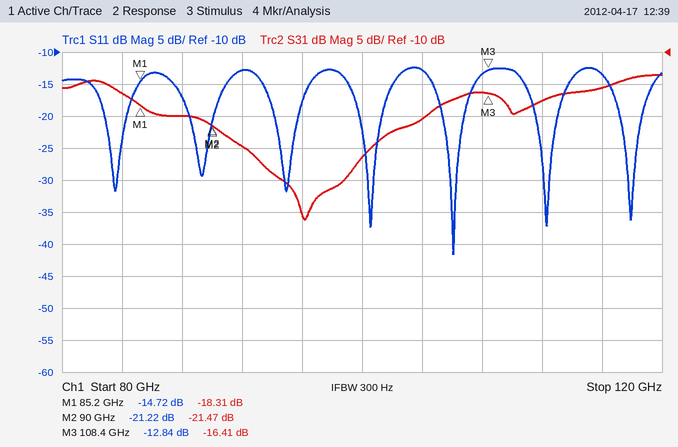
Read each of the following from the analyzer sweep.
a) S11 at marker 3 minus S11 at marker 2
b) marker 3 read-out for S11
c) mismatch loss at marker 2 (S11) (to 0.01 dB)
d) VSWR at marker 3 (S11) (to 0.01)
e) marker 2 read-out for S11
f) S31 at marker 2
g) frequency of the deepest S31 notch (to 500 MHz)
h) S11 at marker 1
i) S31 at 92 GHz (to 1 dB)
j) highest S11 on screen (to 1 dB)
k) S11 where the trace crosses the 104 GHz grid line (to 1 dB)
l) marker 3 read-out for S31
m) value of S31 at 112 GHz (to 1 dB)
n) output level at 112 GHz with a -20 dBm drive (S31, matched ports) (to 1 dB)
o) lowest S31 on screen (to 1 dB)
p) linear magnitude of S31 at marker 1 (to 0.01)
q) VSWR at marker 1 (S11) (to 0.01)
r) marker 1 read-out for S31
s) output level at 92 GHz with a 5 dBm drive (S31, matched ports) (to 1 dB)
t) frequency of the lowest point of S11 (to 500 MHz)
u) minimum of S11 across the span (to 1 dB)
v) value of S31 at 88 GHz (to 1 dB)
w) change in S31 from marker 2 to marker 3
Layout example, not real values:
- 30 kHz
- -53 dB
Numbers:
- 8.38 dB
- -12.84 dB
- 0.03 dB
- 1.59
- -21.22 dB
- -21.47 dB
- 96.0 GHz
- -14.72 dB
- -25 dB
- -12 dB
- -13 dB
- -16.41 dB
- -18 dB
- -38 dBm
- -36 dB
- 0.12
- 1.45
- -18.31 dB
- -20 dBm
- 106.0 GHz
- -42 dB
- -20 dB
- 5.06 dB
